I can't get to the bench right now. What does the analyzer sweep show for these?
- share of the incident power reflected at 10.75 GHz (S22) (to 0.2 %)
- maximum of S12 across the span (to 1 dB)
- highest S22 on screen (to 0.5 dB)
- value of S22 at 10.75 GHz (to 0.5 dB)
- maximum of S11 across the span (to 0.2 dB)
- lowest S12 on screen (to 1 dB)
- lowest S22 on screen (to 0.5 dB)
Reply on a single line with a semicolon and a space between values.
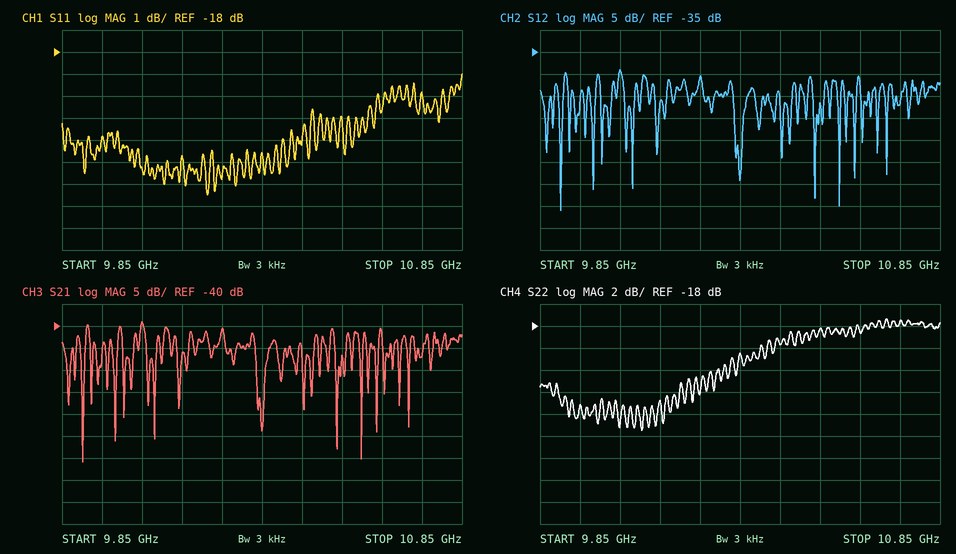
1.8 %; -39 dB; -17.5 dB; -17.5 dB; -19.0 dB; -71 dB; -27.5 dB
